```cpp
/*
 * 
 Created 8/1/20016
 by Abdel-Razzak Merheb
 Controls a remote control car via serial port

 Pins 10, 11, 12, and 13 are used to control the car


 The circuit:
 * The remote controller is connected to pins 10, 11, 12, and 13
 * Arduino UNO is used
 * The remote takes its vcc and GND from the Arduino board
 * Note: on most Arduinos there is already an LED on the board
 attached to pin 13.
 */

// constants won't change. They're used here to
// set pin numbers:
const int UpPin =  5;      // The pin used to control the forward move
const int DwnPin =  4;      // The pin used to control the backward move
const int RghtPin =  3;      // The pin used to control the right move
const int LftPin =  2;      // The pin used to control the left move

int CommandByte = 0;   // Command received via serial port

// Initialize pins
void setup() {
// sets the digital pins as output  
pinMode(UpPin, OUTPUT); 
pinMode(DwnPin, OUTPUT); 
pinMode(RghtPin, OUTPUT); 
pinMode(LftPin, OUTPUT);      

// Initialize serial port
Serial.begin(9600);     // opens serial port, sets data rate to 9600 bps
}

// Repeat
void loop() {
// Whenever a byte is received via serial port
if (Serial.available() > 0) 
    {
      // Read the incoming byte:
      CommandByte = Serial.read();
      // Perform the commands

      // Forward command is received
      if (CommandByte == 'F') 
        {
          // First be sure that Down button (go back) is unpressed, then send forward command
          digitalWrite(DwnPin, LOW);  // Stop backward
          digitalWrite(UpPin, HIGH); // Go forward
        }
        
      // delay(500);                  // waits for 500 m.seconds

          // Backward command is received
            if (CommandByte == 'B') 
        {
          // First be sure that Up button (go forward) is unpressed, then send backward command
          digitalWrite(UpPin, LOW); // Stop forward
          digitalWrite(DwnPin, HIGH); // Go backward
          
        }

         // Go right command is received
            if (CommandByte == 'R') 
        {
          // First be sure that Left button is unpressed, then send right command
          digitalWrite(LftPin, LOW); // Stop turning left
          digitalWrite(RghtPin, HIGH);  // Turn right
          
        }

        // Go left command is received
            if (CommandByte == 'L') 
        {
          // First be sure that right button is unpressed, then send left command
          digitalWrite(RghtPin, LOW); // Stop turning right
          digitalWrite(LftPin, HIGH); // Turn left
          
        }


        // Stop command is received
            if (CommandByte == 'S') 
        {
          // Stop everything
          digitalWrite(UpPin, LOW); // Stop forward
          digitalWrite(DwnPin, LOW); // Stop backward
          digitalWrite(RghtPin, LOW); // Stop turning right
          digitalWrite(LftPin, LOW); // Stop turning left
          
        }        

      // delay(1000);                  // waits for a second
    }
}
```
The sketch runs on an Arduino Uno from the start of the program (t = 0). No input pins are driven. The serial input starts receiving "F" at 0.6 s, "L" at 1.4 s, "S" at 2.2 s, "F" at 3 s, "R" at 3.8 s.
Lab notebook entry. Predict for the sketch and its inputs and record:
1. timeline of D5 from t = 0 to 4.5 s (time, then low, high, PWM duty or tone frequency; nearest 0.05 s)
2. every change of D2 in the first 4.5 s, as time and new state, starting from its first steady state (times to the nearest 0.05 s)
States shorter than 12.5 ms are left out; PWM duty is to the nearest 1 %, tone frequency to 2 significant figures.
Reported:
0 s low; 0.6 s high; 2.2 s low; 3 s high
0 s low; 1.4 s high; 2.2 s low
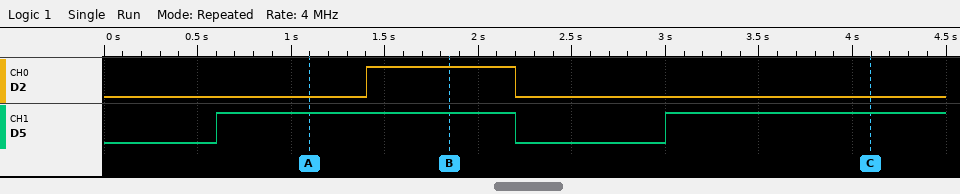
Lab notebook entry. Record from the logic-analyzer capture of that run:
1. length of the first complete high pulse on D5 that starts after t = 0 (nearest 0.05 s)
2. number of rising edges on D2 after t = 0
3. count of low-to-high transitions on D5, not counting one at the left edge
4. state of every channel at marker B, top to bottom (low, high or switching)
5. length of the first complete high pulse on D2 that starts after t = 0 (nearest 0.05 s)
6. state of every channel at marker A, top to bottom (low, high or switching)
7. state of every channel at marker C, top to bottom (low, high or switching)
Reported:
1.60 s
1
2
D2 high, D5 high
0.80 s
D2 low, D5 high
D2 low, D5 high
